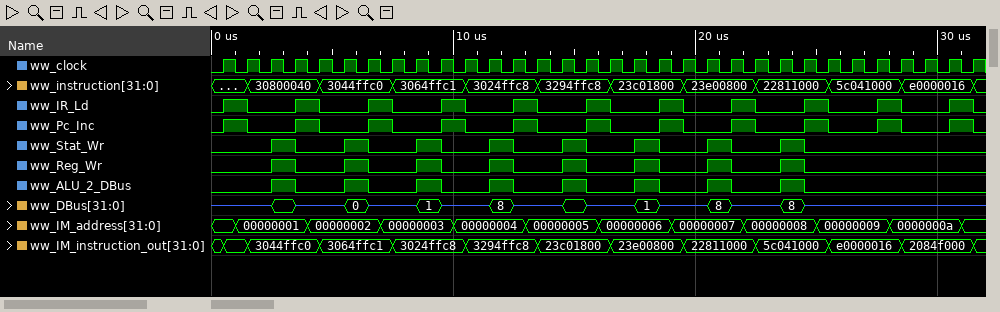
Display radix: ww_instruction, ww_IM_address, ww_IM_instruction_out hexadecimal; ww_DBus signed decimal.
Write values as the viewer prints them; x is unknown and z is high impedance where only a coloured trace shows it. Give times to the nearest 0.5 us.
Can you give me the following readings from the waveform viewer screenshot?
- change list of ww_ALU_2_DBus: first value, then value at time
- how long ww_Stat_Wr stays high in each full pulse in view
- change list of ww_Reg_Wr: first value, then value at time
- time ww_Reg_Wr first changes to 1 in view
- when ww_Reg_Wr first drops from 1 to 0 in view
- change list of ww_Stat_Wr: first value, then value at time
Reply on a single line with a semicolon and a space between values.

0, 1 at 2.5 us, 0 at 3.5 us, 1 at 5.5 us, 0 at 6.5 us, 1 at 8.5 us, 0 at 9.5 us, 1 at 11.5 us, 0 at 12.5 us, 1 at 14.5 us, 0 at 15.5 us, 1 at 17.5 us, 0 at 18.5 us, 1 at 20.5 us, 0 at 21.5 us, 1 at 23.5 us, 0 at 24.5 us; 1 us, 1 us, 1 us, 1 us, 1 us, 1 us, 1 us, 1 us; 0, 1 at 2.5 us, 0 at 3.5 us, 1 at 5.5 us, 0 at 6.5 us, 1 at 8.5 us, 0 at 9.5 us, 1 at 11.5 us, 0 at 12.5 us, 1 at 14.5 us, 0 at 15.5 us, 1 at 17.5 us, 0 at 18.5 us, 1 at 20.5 us, 0 at 21.5 us, 1 at 23.5 us, 0 at 24.5 us; 2.5 us; 3.5 us; 0, 1 at 2.5 us, 0 at 3.5 us, 1 at 5.5 us, 0 at 6.5 us, 1 at 8.5 us, 0 at 9.5 us, 1 at 11.5 us, 0 at 12.5 us, 1 at 14.5 us, 0 at 15.5 us, 1 at 17.5 us, 0 at 18.5 us, 1 at 20.5 us, 0 at 21.5 us, 1 at 23.5 us, 0 at 24.5 us
